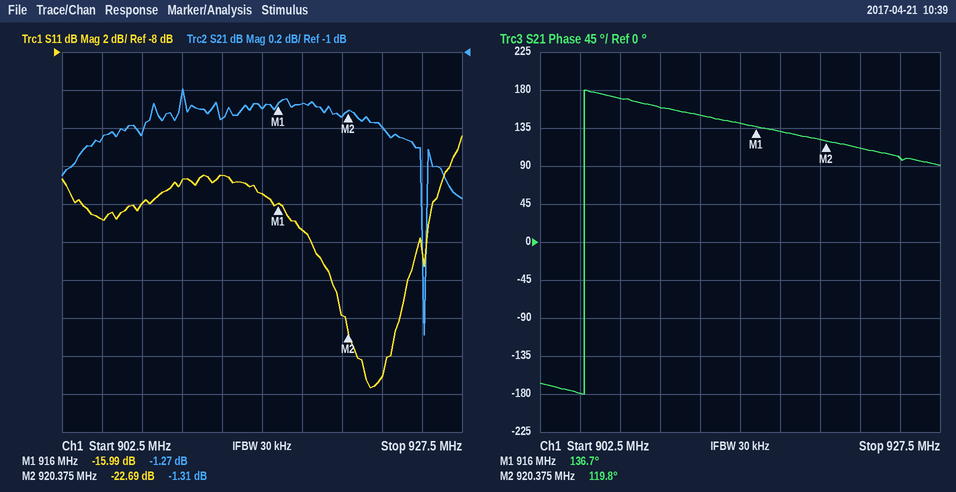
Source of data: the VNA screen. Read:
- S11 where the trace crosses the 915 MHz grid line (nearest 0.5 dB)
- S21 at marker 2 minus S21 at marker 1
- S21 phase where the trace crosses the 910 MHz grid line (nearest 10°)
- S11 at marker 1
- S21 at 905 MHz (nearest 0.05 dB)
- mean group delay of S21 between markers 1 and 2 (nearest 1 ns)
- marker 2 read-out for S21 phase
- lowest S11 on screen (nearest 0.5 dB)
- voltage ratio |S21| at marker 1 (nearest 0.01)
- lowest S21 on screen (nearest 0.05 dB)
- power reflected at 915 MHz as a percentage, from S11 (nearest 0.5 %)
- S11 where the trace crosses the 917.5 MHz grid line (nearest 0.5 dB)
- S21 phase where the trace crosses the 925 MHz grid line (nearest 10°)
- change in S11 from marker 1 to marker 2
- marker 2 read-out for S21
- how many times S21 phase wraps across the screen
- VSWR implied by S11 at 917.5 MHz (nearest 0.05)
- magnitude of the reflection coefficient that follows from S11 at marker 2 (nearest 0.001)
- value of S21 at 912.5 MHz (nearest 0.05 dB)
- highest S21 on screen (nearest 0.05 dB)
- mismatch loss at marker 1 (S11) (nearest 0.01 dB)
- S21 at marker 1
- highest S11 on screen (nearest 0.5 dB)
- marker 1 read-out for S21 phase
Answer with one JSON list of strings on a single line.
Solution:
["-15.5 dB", "-0.04 dB", "160°", "-15.99 dB", "-1.45 dB", "11 ns", "119.8°", "-25.5 dB", "0.86", "-2.50 dB", "3.0 %", "-17.5 dB", "100°", "-6.70 dB", "-1.31 dB", "1", "1.30", "0.073", "-1.35 dB", "-1.20 dB", "0.11 dB", "-1.27 dB", "-12.5 dB", "136.7°"]
